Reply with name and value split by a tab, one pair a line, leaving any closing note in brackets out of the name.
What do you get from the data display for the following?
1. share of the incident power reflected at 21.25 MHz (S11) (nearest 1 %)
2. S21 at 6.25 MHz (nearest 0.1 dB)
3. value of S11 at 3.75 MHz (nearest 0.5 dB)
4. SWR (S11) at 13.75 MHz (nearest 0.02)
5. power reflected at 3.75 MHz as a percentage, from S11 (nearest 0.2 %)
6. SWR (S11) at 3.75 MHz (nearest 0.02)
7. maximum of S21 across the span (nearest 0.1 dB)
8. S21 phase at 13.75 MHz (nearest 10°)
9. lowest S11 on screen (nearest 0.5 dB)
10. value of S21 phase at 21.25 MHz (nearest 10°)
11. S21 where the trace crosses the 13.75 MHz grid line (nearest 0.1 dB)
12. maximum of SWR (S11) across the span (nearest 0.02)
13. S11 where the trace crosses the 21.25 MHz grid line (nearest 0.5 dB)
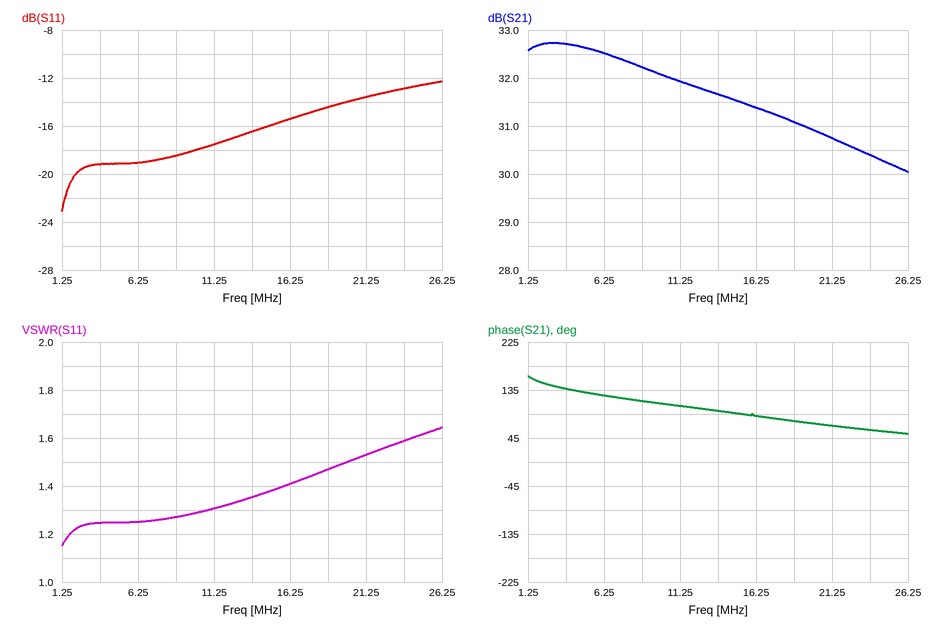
share of the incident power reflected at 21.25 MHz (S11)	4 %
S21 at 6.25 MHz	32.5 dB
value of S11 at 3.75 MHz	-19.0 dB
SWR (S11) at 13.75 MHz	1.36
power reflected at 3.75 MHz as a percentage, from S11	1.2 %
SWR (S11) at 3.75 MHz	1.24
maximum of S21 across the span	32.7 dB
S21 phase at 13.75 MHz	100°
lowest S11 on screen	-23.0 dB
value of S21 phase at 21.25 MHz	70°
S21 where the trace crosses the 13.75 MHz grid line	31.7 dB
maximum of SWR (S11) across the span	1.64
S11 where the trace crosses the 21.25 MHz grid line	-13.5 dB
